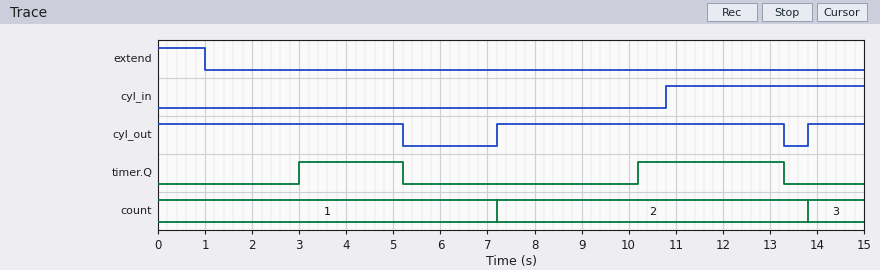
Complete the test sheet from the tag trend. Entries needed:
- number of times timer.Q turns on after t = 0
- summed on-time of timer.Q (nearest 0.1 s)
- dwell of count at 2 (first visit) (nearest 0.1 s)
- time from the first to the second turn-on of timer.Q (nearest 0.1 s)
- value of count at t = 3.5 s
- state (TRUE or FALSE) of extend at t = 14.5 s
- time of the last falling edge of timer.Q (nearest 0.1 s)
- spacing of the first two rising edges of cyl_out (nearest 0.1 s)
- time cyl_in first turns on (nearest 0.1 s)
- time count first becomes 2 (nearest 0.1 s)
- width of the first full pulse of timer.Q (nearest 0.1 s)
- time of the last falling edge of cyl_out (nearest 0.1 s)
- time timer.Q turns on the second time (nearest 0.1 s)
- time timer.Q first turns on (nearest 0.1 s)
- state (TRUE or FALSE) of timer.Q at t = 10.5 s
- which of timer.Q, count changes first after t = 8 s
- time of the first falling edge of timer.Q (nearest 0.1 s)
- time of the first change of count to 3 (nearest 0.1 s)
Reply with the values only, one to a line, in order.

2
5.3 s
6.6 s
7.2 s
1
FALSE
13.3 s
6.6 s
10.8 s
7.2 s
2.2 s
13.3 s
10.2 s
3.0 s
TRUE
timer.Q
5.2 s
13.8 s
